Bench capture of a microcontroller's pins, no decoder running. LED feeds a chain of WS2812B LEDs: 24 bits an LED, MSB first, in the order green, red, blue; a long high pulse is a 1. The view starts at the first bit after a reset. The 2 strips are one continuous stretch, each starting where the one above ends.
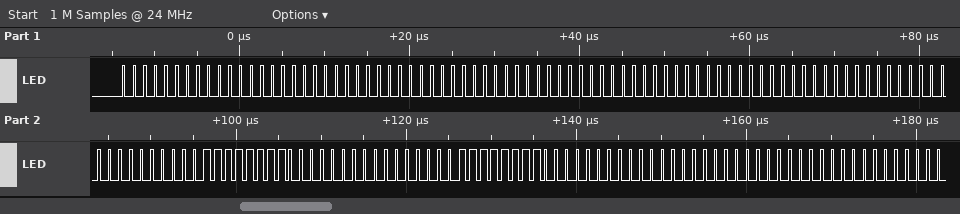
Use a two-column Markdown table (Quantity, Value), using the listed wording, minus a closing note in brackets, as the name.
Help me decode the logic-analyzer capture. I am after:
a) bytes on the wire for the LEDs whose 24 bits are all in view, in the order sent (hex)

| Quantity | Value |
|---|---|
| bytes on the wire for the LEDs whose 24 bits are all in view, in the order sent | 00 00 00 00 00 00 00 00 00 00 00 FF 00 00 FF 00 00 00 |
